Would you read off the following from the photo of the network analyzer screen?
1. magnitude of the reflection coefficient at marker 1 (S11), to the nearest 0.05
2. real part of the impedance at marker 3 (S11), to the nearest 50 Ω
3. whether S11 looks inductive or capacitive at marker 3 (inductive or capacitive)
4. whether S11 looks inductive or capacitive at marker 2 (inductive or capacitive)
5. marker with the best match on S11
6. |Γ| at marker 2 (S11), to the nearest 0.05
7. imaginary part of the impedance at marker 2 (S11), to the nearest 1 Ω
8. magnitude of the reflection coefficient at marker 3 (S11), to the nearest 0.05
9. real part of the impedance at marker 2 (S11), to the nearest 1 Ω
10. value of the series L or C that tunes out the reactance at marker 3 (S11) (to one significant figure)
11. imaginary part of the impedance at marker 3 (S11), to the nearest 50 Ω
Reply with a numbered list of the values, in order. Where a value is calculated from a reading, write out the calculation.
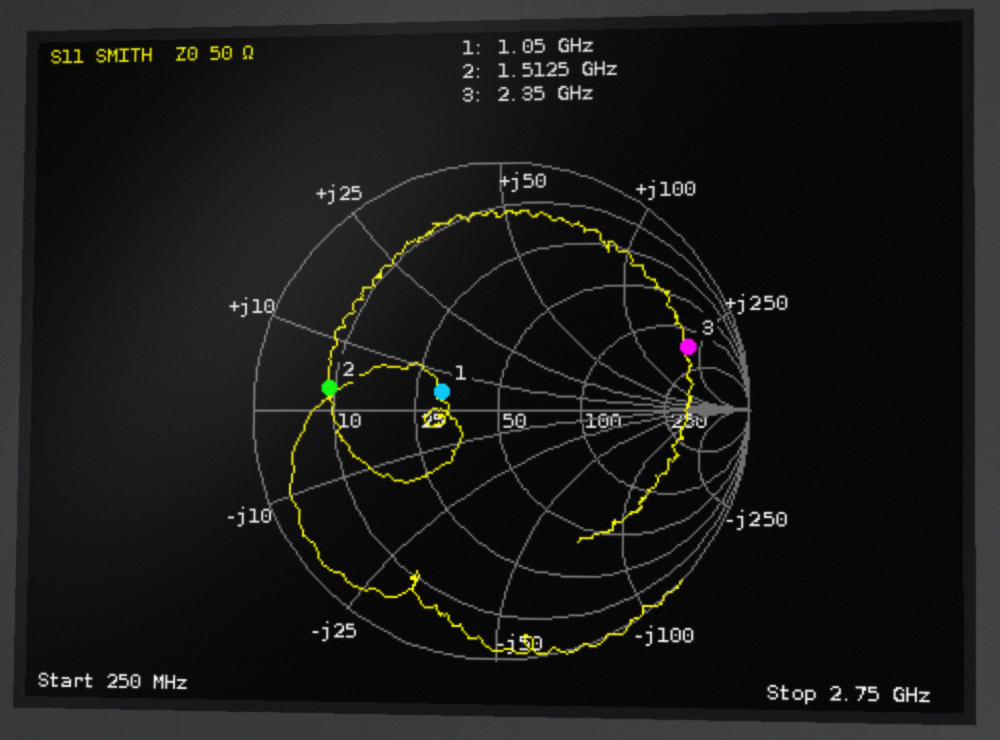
1. 0.25
2. 150 Ω
3. inductive
4. inductive
5. marker 1
6. 0.70
7. +3 Ω
8. 0.80
9. 9 Ω
10. C = 1/(2π × 2.35 GHz × 200 Ω) ≈ 339 fF, so 300 fF to one significant figure
11. +200 Ω
